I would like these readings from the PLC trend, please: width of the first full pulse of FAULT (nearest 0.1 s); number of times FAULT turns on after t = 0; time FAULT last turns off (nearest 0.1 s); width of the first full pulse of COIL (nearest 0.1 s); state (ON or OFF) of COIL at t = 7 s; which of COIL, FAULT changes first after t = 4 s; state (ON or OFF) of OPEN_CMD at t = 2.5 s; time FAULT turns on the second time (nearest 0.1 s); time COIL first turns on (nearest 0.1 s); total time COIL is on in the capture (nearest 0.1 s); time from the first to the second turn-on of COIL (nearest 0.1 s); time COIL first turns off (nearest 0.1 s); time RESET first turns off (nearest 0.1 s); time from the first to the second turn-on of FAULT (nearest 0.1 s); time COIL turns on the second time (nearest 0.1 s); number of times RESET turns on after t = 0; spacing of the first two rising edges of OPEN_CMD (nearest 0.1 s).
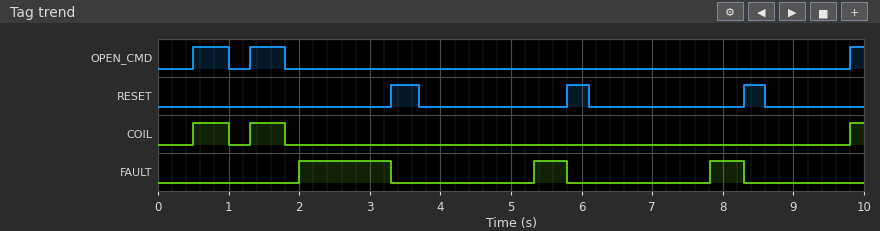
1.3 s
3
8.3 s
0.5 s
OFF
FAULT
OFF
5.3 s
0.5 s
1.2 s
0.8 s
1.0 s
3.7 s
3.3 s
1.3 s
3
0.8 s
